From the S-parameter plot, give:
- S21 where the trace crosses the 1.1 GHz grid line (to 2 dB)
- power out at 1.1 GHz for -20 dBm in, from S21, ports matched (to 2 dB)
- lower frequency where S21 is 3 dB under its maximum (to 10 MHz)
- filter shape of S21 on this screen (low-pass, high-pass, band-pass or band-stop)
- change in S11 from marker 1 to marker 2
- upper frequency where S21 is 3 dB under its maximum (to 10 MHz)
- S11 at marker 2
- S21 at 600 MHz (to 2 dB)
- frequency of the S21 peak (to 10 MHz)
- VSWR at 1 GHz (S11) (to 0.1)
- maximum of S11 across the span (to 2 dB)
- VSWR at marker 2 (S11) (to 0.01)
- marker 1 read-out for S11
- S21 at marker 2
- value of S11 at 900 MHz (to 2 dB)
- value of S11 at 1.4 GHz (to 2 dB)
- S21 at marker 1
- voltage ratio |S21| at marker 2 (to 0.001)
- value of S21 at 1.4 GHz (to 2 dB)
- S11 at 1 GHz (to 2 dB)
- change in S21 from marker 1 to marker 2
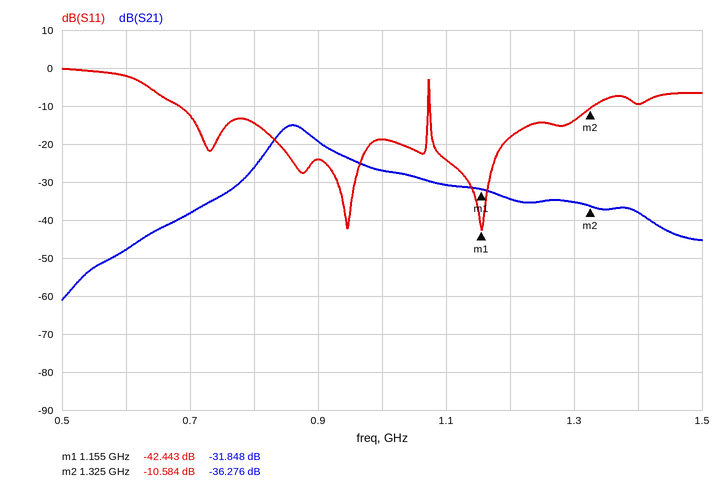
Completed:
-30 dB
-50 dBm
840 MHz
band-pass
31.859 dB
890 MHz
-10.584 dB
-48 dB
860 MHz
1.3
0 dB
1.84
-42.443 dB
-36.276 dB
-24 dB
-10 dB
-31.848 dB
0.015
-38 dB
-18 dB
-4.428 dB
